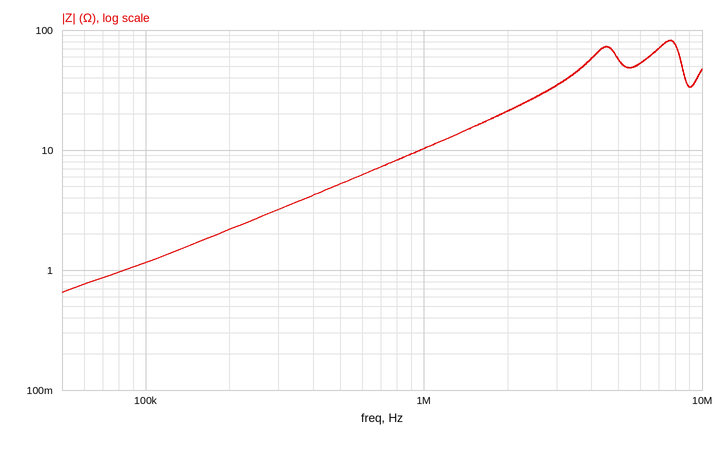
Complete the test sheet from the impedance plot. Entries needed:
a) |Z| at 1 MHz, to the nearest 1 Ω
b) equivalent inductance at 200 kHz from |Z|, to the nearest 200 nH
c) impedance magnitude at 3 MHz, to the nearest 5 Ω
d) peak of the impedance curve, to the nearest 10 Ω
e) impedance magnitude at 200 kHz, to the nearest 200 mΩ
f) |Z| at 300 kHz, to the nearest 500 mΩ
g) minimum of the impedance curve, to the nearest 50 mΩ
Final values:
10 Ω
1.8 µH
35 Ω
80 Ω
2.2 Ω
3.0 Ω
650 mΩ
